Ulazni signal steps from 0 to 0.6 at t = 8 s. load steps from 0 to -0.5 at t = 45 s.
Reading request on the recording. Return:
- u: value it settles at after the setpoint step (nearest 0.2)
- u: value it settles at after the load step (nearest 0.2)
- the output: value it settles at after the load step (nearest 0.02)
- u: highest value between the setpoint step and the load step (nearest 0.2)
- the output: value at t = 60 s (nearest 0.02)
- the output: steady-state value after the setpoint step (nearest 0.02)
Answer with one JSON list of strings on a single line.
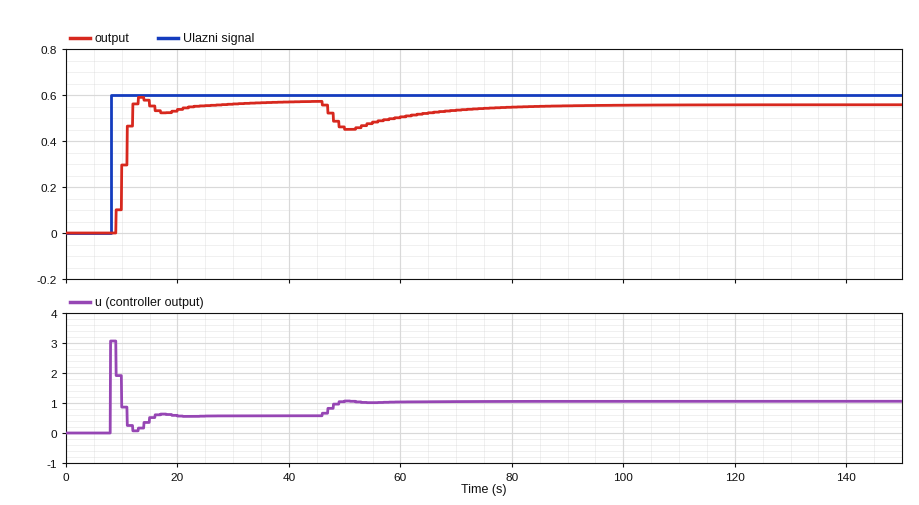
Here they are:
["0.6", "1.0", "0.56", "3.0", "0.50", "0.58"]
